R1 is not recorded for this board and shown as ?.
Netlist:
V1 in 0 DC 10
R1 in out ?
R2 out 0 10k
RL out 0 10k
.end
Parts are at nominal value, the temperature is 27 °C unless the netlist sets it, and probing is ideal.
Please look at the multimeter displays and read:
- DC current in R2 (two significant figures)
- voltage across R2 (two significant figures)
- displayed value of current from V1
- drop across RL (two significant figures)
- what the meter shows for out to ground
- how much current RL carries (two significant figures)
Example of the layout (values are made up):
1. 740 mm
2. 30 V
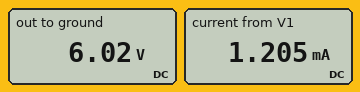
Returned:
1. 600 µA
2. 6.0 V
3. 1.205 mA
4. 6.0 V
5. 6.02 V
6. 600 µA
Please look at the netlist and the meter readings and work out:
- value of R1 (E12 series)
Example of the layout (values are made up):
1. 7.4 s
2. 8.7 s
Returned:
1. 3.3 kΩ
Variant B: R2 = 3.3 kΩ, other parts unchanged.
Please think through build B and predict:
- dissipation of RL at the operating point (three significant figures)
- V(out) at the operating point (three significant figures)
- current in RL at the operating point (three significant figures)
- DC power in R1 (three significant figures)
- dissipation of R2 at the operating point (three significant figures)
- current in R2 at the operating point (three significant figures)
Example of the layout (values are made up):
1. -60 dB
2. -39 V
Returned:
1. 1.84 mW
2. 4.29 V
3. 429 µA
4. 9.87 mW
5. 5.58 mW
6. 1.30 mA
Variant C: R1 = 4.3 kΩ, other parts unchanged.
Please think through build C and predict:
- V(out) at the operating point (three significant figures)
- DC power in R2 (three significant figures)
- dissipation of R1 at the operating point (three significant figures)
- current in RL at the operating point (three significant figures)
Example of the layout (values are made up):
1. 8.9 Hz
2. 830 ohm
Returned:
1. 5.38 V
2. 2.89 mW
3. 4.97 mW
4. 538 µA
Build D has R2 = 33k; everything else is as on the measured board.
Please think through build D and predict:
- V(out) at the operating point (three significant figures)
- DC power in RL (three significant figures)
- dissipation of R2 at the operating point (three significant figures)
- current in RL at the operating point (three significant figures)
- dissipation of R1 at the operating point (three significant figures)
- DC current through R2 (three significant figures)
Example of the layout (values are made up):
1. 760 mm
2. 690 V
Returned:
1. 6.99 V
2. 4.89 mW
3. 1.48 mW
4. 699 µA
5. 2.74 mW
6. 212 µA
